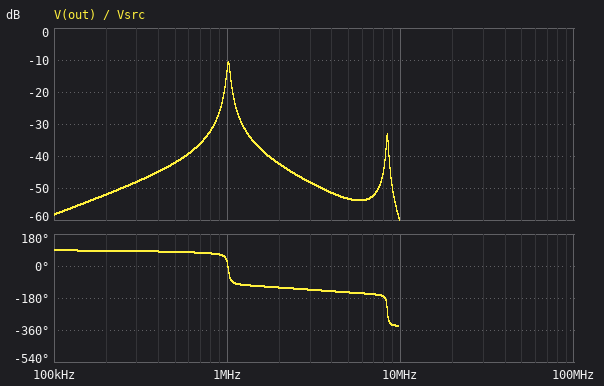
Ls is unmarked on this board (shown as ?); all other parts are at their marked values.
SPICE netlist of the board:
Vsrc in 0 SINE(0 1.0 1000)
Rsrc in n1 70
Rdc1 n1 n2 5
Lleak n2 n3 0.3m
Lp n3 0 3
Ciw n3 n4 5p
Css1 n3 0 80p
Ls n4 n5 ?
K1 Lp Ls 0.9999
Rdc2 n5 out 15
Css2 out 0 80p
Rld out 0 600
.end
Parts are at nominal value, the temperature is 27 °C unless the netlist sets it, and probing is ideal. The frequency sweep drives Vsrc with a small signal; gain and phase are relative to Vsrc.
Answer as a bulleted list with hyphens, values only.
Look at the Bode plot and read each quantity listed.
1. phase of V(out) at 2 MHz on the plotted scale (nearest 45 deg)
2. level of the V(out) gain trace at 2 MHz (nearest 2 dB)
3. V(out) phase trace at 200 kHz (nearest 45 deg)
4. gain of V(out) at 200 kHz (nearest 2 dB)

- -135 deg
- -42 dB
- 90 deg
- -52 dB
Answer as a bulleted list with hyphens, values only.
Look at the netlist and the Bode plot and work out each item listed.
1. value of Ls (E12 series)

- 390 mH
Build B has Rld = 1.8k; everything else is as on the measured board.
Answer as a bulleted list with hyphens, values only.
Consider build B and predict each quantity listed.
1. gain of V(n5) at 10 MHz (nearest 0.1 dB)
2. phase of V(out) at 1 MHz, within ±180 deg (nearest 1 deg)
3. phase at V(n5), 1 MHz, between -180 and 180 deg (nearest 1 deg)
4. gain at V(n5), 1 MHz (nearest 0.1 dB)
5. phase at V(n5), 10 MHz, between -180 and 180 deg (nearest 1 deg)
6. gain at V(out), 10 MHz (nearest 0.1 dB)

- -60.5 dB
- -8 deg
- -7 deg
- -5.2 dB
- 12 deg
- -60.6 dB
